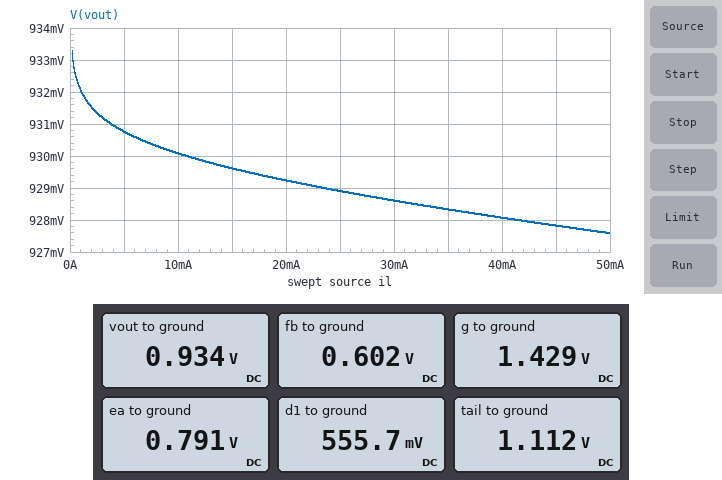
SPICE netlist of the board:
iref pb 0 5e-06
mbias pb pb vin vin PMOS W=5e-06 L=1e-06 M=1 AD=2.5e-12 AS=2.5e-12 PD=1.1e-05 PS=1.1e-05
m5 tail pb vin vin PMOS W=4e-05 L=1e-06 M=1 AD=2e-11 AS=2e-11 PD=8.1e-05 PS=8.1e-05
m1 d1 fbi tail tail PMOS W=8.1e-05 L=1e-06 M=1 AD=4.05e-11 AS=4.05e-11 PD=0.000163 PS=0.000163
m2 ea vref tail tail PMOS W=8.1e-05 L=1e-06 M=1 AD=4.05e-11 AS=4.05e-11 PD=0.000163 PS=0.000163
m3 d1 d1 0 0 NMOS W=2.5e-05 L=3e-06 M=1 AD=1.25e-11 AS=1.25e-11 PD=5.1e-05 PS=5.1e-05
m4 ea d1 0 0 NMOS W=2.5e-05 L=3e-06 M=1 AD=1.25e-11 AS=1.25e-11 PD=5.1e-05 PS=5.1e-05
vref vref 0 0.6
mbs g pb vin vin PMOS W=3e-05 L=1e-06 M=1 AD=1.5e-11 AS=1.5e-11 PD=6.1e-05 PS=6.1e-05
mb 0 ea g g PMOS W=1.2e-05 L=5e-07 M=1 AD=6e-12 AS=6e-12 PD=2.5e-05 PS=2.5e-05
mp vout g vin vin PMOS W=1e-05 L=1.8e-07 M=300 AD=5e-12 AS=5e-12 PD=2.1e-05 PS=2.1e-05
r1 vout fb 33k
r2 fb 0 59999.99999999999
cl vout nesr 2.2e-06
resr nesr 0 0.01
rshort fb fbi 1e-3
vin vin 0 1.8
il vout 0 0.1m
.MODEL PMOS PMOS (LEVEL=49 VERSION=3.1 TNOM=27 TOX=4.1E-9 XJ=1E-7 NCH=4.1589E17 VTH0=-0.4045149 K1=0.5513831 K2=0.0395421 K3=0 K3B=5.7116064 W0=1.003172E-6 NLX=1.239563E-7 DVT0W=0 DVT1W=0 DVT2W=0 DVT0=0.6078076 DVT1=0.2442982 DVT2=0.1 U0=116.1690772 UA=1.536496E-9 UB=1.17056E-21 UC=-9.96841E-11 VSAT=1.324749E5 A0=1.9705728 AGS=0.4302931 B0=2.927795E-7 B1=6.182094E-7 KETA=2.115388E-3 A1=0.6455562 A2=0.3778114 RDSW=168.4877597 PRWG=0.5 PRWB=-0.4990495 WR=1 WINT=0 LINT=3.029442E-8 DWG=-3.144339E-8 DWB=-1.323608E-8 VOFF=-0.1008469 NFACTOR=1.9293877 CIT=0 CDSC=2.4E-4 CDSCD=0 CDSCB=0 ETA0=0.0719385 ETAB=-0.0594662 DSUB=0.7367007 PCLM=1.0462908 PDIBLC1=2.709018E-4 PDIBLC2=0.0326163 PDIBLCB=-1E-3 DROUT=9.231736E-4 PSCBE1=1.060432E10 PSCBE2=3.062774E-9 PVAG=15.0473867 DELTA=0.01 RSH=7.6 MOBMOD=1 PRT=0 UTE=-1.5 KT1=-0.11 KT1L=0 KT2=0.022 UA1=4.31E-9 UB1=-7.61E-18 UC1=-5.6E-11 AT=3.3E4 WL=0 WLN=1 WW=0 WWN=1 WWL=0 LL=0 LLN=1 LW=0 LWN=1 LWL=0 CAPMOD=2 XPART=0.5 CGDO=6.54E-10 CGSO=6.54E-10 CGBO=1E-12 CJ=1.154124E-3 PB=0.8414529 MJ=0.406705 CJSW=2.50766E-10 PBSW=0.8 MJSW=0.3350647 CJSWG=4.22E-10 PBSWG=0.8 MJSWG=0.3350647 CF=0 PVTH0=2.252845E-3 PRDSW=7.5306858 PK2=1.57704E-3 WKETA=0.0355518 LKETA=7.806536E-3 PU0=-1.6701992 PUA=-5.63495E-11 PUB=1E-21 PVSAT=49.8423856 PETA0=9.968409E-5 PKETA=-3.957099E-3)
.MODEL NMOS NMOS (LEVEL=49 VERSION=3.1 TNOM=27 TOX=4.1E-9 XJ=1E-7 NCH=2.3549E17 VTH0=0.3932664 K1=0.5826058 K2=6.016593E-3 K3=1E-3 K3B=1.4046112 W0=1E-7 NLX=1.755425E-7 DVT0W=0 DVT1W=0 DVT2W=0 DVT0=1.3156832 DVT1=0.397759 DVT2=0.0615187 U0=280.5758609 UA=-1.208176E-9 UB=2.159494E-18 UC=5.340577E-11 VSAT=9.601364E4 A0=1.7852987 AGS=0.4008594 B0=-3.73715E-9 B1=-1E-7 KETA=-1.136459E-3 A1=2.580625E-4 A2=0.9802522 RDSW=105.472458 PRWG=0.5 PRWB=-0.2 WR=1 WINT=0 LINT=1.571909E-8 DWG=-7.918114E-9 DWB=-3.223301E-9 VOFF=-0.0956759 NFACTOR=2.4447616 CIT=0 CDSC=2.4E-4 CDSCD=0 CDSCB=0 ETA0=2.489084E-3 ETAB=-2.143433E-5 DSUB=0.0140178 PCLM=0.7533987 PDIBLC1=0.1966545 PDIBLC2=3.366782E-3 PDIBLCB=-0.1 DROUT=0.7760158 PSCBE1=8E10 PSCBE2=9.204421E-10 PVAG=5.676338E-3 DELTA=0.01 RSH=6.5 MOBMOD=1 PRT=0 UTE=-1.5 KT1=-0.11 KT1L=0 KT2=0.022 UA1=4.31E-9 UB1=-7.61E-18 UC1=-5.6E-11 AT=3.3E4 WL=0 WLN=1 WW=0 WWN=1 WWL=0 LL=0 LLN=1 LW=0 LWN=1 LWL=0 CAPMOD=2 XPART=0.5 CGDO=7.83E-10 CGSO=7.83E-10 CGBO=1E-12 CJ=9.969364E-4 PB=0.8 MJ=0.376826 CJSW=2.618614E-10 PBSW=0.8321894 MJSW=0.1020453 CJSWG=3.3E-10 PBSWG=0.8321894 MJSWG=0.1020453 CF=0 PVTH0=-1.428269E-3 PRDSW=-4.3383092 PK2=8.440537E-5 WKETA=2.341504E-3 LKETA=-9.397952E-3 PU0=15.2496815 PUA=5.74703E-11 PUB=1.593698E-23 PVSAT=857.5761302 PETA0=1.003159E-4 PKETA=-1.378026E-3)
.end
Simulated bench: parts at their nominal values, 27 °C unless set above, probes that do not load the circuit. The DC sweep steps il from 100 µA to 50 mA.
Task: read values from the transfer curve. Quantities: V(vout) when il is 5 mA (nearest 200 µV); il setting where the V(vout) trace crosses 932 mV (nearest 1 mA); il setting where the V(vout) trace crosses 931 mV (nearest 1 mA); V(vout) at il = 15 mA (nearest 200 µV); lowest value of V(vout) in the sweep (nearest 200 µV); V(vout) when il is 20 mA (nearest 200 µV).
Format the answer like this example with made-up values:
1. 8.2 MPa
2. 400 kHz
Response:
1. 930.8 mV
2. 1 mA
3. 4 mA
4. 929.6 mV
5. 927.6 mV
6. 929.2 mV
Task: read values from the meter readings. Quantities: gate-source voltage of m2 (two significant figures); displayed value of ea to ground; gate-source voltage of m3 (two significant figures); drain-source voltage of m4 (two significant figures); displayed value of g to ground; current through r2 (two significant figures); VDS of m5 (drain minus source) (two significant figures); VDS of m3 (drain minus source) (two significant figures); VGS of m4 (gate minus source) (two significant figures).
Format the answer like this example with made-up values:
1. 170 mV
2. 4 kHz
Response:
1. -510 mV
2. 0.791 V
3. 560 mV
4. 790 mV
5. 1.429 V
6. 10 µA
7. -690 mV
8. 560 mV
9. 560 mV
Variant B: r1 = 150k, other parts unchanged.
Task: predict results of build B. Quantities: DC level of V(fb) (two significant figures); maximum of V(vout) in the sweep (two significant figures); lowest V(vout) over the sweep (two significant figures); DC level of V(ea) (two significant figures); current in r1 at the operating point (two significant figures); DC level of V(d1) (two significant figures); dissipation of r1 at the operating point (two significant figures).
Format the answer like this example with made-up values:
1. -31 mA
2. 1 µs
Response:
1. 510 mV
2. 1.8 V
3. 1.7 V
4. 22 mV
5. 8.6 µA
6. 600 mV
7. 11 µW
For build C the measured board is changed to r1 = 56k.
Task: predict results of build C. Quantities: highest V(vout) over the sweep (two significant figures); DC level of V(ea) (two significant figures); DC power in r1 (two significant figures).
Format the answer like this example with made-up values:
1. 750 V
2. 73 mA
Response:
1. 1.2 V
2. 780 mV
3. 5.6 µW
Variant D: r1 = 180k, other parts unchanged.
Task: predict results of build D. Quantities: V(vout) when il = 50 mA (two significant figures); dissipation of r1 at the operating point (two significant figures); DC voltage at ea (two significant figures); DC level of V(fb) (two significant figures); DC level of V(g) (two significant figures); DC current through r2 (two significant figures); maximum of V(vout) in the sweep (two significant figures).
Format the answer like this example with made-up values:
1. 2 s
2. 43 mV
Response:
1. 1.7 V
2. 10 µW
3. 6.1 mV
4. 450 mV
5. 660 mV
6. 7.5 µA
7. 1.8 V
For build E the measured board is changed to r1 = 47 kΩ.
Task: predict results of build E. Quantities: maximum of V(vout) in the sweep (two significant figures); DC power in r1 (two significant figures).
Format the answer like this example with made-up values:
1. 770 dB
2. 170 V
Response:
1. 1.1 V
2. 4.7 µW
